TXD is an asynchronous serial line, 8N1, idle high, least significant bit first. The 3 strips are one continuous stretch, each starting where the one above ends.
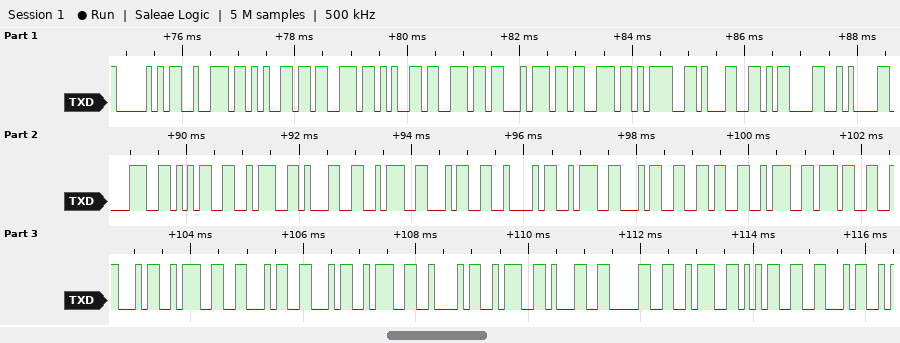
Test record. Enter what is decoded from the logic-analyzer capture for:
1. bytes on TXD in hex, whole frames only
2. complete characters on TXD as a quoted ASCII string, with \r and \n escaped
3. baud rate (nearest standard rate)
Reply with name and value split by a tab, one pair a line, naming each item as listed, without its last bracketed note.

bytes on TXD in hex, whole frames only	0x50 0x72 0x65 0x73 0x65 0x6E 0x74 0x73 0x3D 0x31 0x0D 0x0A 0x38 0x35 0x3A 0x31 0x3A 0x34 0x42 0x3A 0x34 0x36 0x3A 0x37 0x46 0x3A 0x46 0x46 0x3A 0x42 0x3A 0x31 0x30 0x3A 0x35 0x46
complete characters on TXD as a quoted ASCII string, with \r and \n escaped	"Presents=1\r\n85:1:4B:46:7F:FF:B:10:5F"
baud rate	9600 baud
